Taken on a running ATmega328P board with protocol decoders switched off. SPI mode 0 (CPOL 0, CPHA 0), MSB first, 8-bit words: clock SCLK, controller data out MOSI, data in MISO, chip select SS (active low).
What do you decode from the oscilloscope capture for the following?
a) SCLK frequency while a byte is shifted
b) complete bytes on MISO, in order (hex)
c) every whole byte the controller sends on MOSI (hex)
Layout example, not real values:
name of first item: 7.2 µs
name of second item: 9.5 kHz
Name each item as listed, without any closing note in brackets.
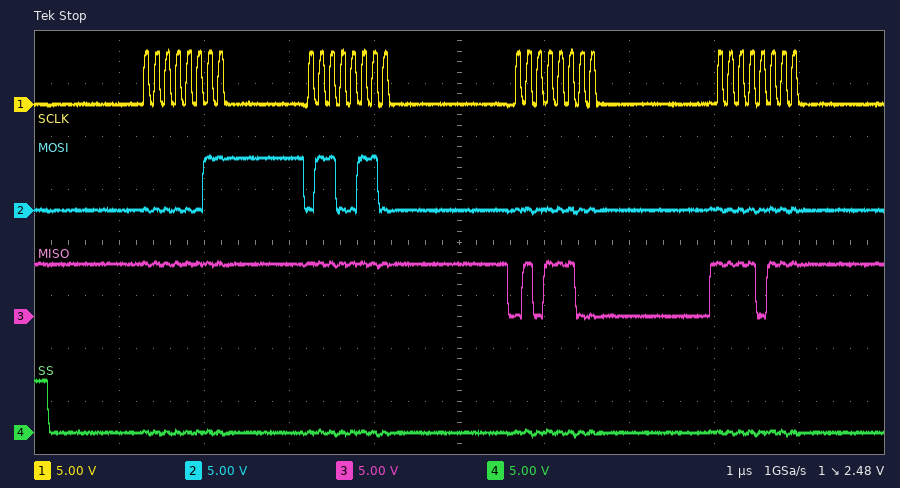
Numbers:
SCLK frequency while a byte is shifted: 8 MHz
complete bytes on MISO, in order: FF FF 5C F7
every whole byte the controller sends on MOSI: 03 66 00 00
